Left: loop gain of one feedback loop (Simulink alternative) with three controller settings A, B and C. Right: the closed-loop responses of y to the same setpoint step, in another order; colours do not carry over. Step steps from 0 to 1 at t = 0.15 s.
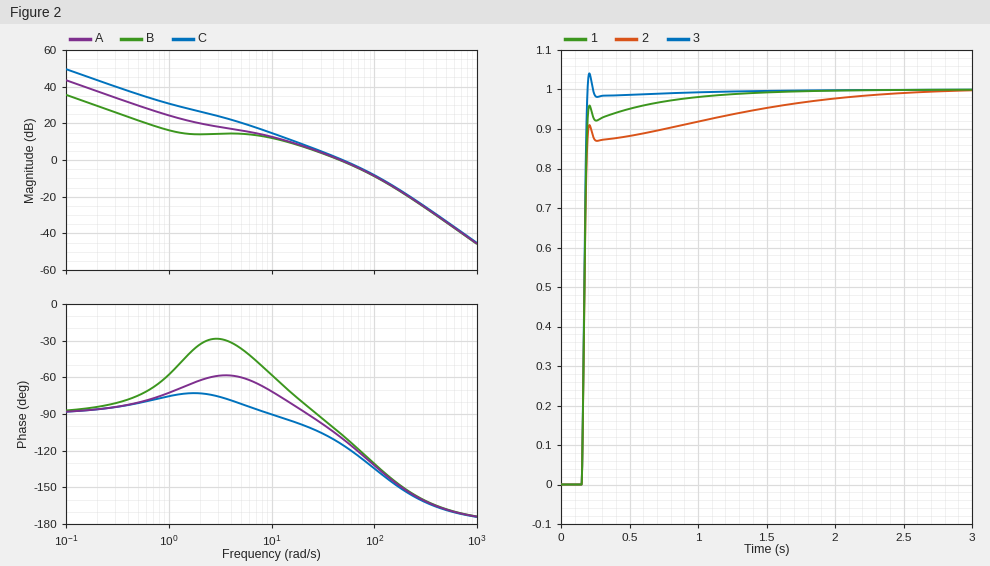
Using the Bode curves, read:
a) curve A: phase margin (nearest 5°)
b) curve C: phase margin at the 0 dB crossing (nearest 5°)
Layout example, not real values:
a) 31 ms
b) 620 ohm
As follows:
a) 70°
b) 65°
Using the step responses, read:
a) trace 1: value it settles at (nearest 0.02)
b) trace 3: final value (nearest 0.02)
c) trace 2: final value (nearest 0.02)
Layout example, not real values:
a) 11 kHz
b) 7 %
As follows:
a) 1.00
b) 1.00
c) 1.00
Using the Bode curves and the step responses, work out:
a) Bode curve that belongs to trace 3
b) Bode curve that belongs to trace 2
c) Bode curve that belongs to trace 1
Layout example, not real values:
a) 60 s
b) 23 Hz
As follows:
a) C
b) B
c) A
